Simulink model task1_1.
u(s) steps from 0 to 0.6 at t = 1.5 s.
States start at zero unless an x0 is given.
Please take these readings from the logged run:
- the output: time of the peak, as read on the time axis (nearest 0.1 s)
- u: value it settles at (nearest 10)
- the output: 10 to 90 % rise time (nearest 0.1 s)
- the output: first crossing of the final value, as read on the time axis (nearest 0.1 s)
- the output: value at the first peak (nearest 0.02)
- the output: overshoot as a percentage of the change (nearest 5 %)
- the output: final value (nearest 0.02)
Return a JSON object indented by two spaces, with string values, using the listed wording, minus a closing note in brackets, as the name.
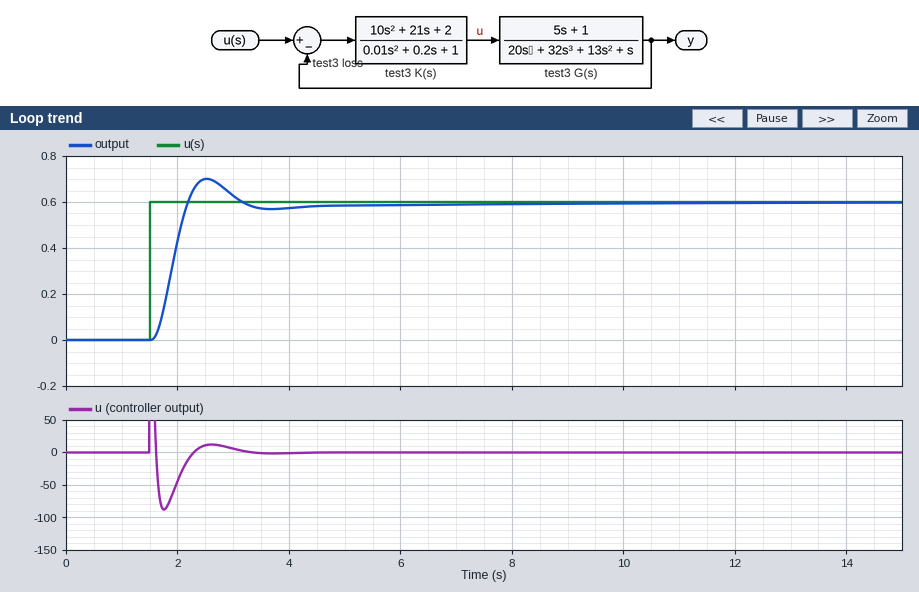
{
  "the output: time of the peak, as read on the time axis": "2.5 s",
  "u: value it settles at": "0",
  "the output: 10 to 90 % rise time": "0.4 s",
  "the output: first crossing of the final value, as read on the time axis": "2.2 s",
  "the output: value at the first peak": "0.70",
  "the output: overshoot as a percentage of the change": "15 %",
  "the output: final value": "0.60"
}
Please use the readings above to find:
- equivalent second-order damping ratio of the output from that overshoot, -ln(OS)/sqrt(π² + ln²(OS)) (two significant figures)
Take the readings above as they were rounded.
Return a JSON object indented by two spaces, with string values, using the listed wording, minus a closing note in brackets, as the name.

{
  "equivalent second-order damping ratio of the output from that overshoot, -ln(OS)/sqrt(π² + ln²(OS))": "0.52"
}
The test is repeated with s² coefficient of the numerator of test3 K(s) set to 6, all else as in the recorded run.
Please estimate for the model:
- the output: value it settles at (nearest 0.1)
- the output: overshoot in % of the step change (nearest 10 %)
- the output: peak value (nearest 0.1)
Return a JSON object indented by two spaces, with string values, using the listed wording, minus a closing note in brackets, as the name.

{
  "the output: value it settles at": "0.6",
  "the output: overshoot in % of the step change": "30 %",
  "the output: peak value": "0.8"
}
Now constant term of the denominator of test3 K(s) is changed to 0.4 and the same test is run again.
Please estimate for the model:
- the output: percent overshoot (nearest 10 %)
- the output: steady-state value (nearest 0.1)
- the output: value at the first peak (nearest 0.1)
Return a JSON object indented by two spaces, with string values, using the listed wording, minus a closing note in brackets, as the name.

{
  "the output: percent overshoot": "70 %",
  "the output: steady-state value": "0.6",
  "the output: value at the first peak": "1.0"
}
